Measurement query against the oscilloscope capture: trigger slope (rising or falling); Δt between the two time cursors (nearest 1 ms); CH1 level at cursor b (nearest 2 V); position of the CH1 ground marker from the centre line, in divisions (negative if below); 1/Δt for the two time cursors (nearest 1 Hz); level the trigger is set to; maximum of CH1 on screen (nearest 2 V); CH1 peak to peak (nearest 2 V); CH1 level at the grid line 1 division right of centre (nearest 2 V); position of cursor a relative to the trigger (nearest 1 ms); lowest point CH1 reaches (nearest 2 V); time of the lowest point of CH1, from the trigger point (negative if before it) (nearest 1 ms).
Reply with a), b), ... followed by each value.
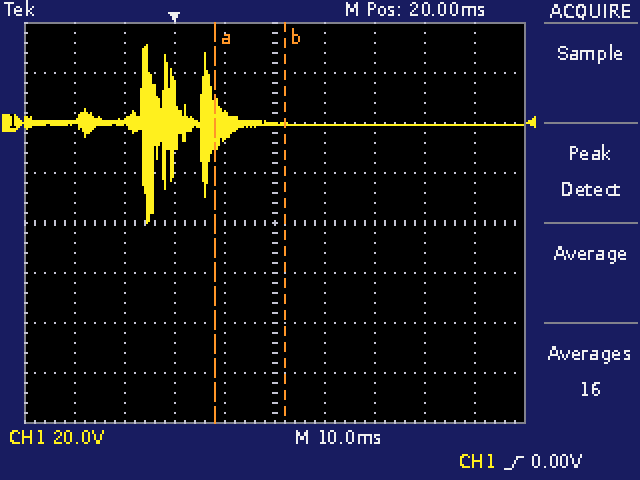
a) rising
b) 14 ms
c) 0 V
d) +2.0 div
e) 71 Hz
f) 0.00 V
g) 32 V
h) 72 V
i) 0 V
j) +8 ms
k) -40 V
l) -5 ms
